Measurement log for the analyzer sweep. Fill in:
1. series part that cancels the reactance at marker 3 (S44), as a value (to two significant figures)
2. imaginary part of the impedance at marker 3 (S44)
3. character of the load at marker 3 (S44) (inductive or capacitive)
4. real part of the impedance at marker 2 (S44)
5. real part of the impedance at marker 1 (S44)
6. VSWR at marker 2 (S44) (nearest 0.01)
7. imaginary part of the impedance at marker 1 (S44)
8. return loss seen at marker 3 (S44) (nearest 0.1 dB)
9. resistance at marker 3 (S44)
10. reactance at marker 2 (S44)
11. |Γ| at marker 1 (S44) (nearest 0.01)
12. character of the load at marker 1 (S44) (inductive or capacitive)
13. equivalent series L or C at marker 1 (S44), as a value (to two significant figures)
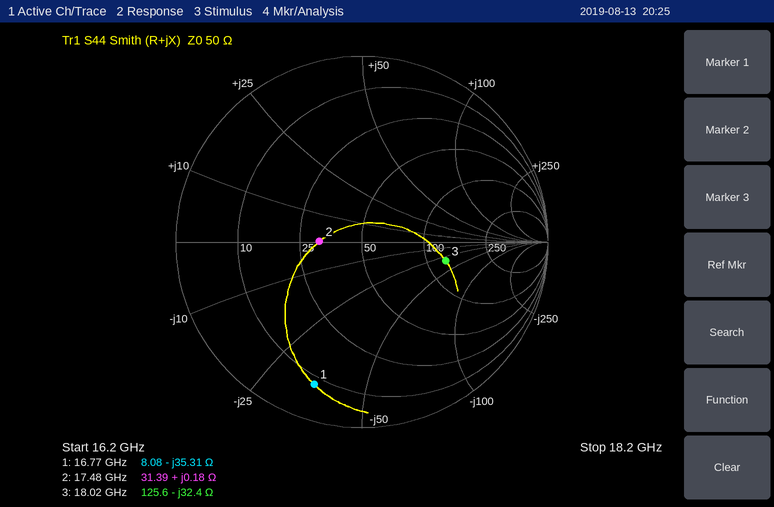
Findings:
290 pH
-32.4 Ω
capacitive
31.39 Ω
8.08 Ω
1.59
-35.31 Ω
6.7 dB
125.6 Ω
+0.18 Ω
0.81
capacitive
270 fF
